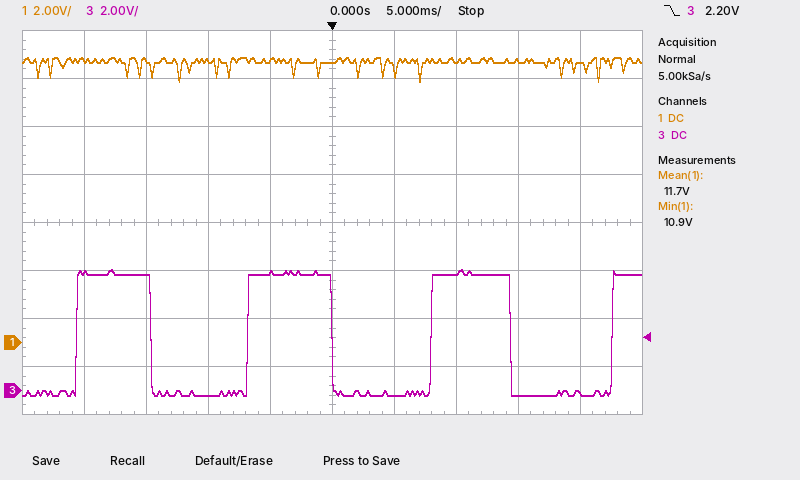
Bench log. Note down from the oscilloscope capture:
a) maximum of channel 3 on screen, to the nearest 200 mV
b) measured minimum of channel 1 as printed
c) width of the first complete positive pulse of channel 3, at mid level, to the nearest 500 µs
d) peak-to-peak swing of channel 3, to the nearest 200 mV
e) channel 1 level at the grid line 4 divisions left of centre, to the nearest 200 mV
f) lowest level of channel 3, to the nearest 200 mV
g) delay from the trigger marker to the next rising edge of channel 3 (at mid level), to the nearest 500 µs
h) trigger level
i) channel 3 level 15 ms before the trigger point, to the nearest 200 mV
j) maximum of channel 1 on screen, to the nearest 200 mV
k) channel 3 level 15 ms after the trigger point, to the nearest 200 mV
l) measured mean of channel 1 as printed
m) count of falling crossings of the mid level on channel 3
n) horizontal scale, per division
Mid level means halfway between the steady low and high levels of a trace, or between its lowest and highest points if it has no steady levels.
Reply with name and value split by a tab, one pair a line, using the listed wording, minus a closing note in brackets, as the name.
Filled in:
maximum of channel 3 on screen, to the nearest 200 mV	5.0 V
measured minimum of channel 1 as printed	10.9 V
width of the first complete positive pulse of channel 3, at mid level, to the nearest 500 µs	6.0 ms
peak-to-peak swing of channel 3, to the nearest 200 mV	5.2 V
channel 1 level at the grid line 4 divisions left of centre, to the nearest 200 mV	11.8 V
lowest level of channel 3, to the nearest 200 mV	-200 mV
delay from the trigger marker to the next rising edge of channel 3 (at mid level), to the nearest 500 µs	8.0 ms
trigger level	2.20 V
channel 3 level 15 ms before the trigger point, to the nearest 200 mV	4.8 V
maximum of channel 1 on screen, to the nearest 200 mV	11.8 V
channel 3 level 15 ms after the trigger point, to the nearest 200 mV	-200 mV
measured mean of channel 1 as printed	11.7 V
count of falling crossings of the mid level on channel 3	3
horizontal scale, per division	5 ms
